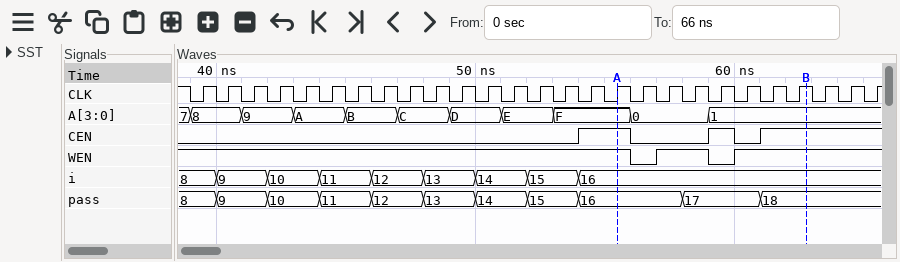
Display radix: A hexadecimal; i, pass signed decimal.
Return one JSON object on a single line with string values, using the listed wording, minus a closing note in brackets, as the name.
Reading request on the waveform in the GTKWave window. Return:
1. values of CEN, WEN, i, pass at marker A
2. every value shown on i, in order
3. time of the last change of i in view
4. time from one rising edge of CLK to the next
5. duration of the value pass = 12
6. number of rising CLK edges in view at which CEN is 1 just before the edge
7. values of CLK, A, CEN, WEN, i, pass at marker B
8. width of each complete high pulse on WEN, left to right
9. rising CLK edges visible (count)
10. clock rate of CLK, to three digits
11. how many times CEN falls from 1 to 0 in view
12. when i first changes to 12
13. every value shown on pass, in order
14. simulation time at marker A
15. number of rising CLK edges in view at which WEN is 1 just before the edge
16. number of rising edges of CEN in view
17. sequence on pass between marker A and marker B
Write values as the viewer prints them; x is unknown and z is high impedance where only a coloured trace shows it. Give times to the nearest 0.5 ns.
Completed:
{"values of CEN, WEN, i, pass at marker A": "CEN=1, WEN=1, i=16, pass=16", "every value shown on i, in order": "8, 9, 10, 11, 12, 13, 14, 15, 16", "time of the last change of i in view": "54 ns", "time from one rising edge of CLK to the next": "1 ns", "duration of the value pass = 12": "2 ns", "number of rising CLK edges in view at which CEN is 1 just before the edge": "8", "values of CLK, A, CEN, WEN, i, pass at marker B": "CLK=1, A=1, CEN=1, WEN=1, i=16, pass=18", "width of each complete high pulse on WEN, left to right": "2 ns", "rising CLK edges visible": "27", "clock rate of CLK, to three digits": "1.00 GHz", "how many times CEN falls from 1 to 0 in view": "2", "when i first changes to 12": "46 ns", "every value shown on pass, in order": "8, 9, 10, 11, 12, 13, 14, 15, 16, 17, 18", "simulation time at marker A": "55.5 ns", "number of rising CLK edges in view at which WEN is 1 just before the edge": "25", "number of rising edges of CEN in view": "3", "sequence on pass between marker A and marker B": "16, 17, 18"}
